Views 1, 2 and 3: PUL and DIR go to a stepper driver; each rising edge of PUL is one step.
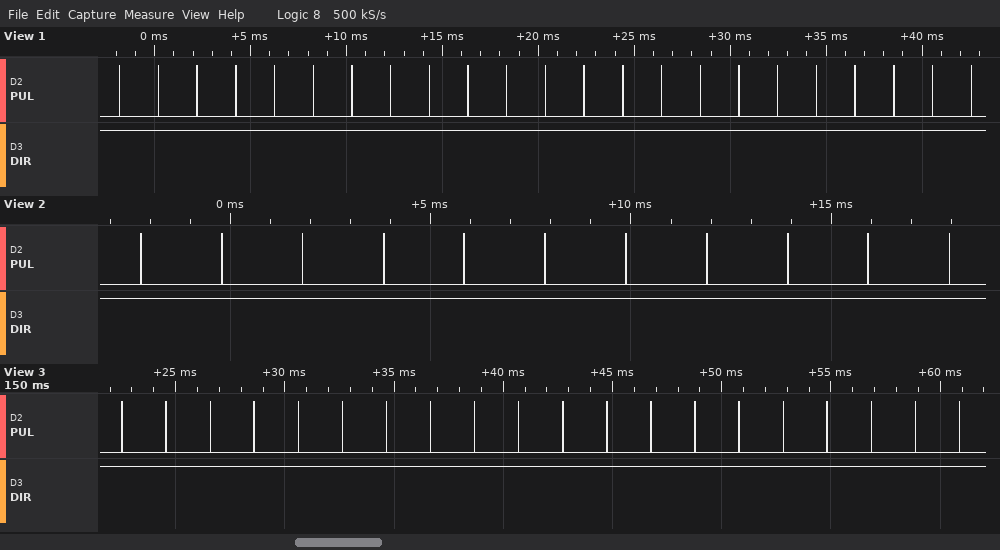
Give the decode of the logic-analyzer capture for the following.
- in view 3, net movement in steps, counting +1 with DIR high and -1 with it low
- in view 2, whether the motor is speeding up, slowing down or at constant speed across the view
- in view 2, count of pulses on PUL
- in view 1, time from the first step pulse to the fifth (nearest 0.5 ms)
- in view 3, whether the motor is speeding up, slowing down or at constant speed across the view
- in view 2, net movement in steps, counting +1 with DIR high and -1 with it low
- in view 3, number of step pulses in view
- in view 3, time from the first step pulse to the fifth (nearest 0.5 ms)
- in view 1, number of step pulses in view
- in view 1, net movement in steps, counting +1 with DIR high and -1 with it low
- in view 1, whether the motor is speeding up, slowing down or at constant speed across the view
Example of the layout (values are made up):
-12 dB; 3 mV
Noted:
+20; constant speed; 11; 8.0 ms; constant speed; +11; 20; 8.0 ms; 23; +23; constant speed
